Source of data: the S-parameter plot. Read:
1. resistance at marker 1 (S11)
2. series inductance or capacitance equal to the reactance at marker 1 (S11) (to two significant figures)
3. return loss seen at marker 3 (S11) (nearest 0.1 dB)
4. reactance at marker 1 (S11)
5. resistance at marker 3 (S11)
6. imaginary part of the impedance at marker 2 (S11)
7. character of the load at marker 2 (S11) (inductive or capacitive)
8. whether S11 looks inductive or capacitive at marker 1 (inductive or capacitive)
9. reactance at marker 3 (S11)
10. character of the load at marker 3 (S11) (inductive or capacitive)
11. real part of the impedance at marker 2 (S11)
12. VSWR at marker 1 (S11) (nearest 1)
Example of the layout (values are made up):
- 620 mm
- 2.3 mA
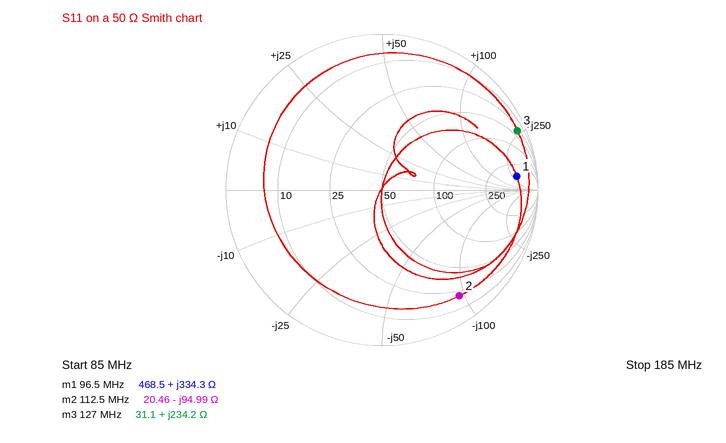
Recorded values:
- 468.5 Ω
- 550 nH
- 0.5 dB
- +334.3 Ω
- 31.1 Ω
- -94.99 Ω
- capacitive
- inductive
- +234.2 Ω
- inductive
- 20.46 Ω
- 14
